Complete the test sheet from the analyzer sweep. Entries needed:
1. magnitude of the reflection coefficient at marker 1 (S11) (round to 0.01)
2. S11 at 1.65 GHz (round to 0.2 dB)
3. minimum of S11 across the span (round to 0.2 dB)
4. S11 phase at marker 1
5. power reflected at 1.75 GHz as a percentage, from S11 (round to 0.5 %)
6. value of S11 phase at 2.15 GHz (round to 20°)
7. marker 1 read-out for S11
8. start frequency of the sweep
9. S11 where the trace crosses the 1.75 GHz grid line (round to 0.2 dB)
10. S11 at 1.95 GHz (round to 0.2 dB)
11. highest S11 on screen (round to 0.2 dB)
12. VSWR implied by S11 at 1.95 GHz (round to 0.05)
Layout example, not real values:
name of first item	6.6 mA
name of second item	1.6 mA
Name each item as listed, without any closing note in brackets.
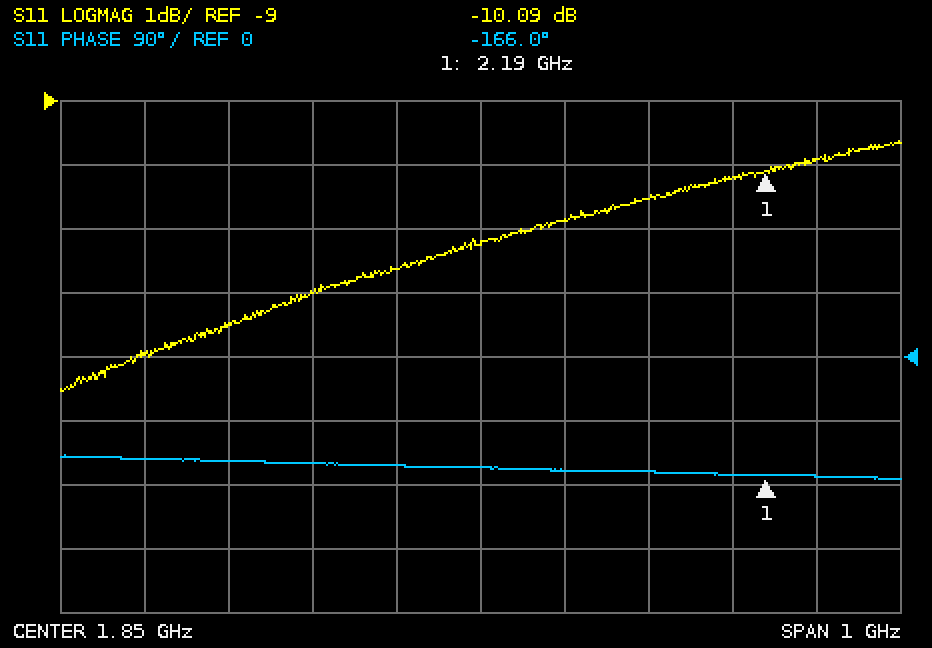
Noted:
magnitude of the reflection coefficient at marker 1 (S11)	0.31
S11 at 1.65 GHz	-12.0 dB
minimum of S11 across the span	-13.6 dB
S11 phase at marker 1	-166.0°
power reflected at 1.75 GHz as a percentage, from S11	7.0 %
value of S11 phase at 2.15 GHz	-160°
marker 1 read-out for S11	-10.09 dB
start frequency of the sweep	1.35 GHz
S11 where the trace crosses the 1.75 GHz grid line	-11.6 dB
S11 at 1.95 GHz	-10.8 dB
highest S11 on screen	-9.6 dB
VSWR implied by S11 at 1.95 GHz	1.80
